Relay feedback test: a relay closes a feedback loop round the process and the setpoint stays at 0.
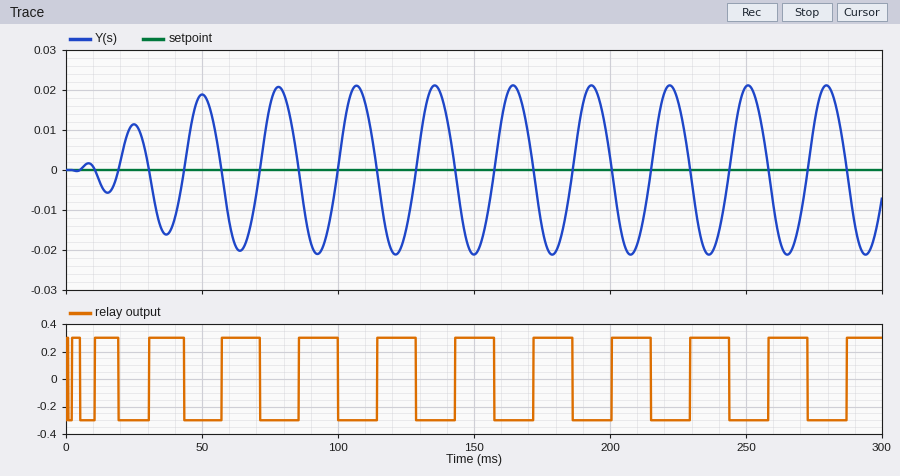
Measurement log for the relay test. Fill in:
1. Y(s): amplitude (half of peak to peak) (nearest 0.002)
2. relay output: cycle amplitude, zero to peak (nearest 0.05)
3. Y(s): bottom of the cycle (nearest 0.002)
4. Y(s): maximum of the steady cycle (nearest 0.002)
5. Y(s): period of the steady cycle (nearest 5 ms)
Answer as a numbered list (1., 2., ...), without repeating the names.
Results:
1. 0.022
2. 0.30
3. -0.022
4. 0.022
5. 30 ms
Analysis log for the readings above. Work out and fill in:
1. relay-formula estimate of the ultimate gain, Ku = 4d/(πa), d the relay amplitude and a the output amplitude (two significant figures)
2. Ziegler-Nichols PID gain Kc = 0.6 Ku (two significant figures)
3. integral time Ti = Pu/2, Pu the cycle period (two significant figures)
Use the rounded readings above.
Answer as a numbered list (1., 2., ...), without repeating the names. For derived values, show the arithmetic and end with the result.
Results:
1. 4 × 0.3 / (π × 0.022) = 17
2. 0.6 × 17 = 10
3. 30 / 2 = 15 ms
